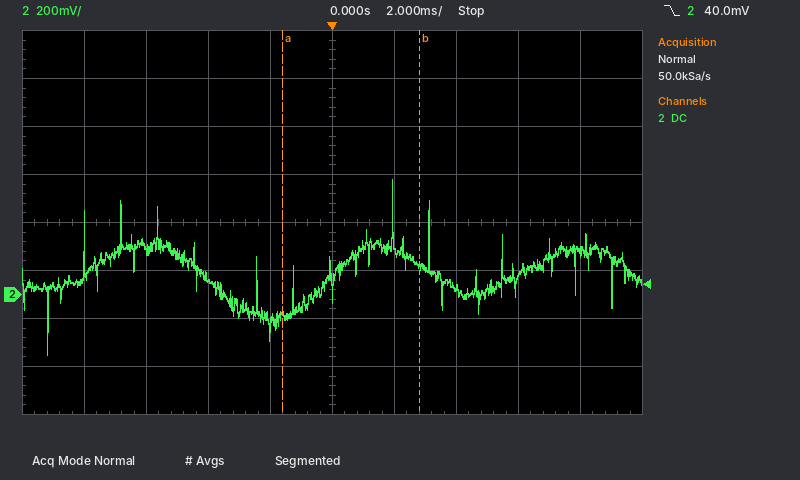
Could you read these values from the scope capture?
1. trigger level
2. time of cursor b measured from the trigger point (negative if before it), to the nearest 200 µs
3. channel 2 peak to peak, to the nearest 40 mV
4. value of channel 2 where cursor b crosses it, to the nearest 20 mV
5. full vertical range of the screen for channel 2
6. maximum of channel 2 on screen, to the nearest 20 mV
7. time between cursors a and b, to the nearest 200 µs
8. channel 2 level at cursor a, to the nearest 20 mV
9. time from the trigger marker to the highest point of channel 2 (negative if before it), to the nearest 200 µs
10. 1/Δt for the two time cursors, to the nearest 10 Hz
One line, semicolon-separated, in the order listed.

40.0 mV; +2.8 ms; 720 mV; 120 mV; 1.6 V; 480 mV; 4.4 ms; -80 mV; +2.0 ms; 230 Hz
